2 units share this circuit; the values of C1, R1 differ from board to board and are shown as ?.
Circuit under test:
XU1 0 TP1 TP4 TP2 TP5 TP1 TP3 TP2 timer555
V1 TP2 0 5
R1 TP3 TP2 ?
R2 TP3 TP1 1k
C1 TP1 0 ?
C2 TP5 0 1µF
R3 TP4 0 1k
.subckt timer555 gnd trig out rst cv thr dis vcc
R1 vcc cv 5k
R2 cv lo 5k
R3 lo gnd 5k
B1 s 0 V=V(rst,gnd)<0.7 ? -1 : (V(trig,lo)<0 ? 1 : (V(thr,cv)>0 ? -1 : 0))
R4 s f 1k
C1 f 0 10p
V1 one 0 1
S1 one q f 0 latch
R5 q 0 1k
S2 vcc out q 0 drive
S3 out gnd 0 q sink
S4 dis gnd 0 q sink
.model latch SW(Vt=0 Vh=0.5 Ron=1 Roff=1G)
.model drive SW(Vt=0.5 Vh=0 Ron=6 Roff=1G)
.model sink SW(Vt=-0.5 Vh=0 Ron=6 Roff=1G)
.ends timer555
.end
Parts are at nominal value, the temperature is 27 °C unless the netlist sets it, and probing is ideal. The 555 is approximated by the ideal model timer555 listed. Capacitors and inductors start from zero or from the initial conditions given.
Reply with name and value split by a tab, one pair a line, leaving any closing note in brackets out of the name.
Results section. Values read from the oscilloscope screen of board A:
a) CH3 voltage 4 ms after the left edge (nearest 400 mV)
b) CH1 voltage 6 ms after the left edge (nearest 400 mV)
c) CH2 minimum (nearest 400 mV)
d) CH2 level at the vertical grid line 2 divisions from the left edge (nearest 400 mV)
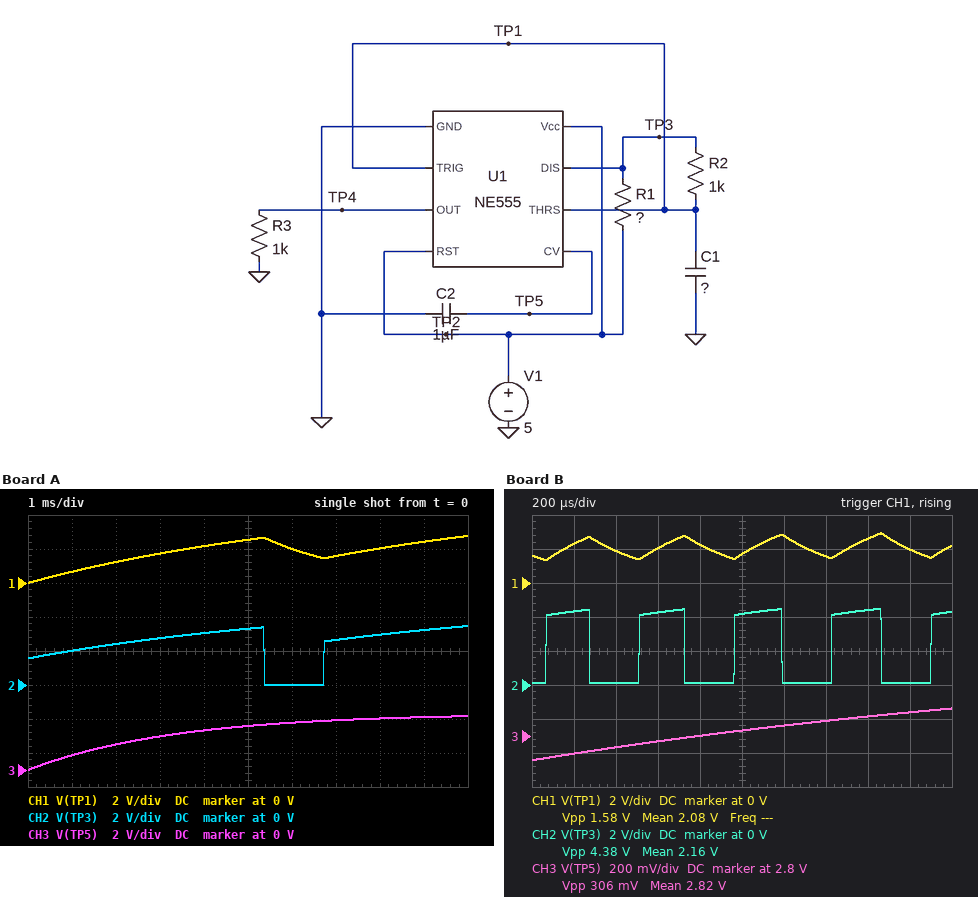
CH3 voltage 4 ms after the left edge	2.4 V
CH1 voltage 6 ms after the left edge	2.0 V
CH2 minimum	0 V
CH2 level at the vertical grid line 2 divisions from the left edge	2.4 V
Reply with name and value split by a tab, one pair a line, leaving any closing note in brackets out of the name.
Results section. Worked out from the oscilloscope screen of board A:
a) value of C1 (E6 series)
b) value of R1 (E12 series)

value of C1	2.2 µF
value of R1	2.2 kΩ
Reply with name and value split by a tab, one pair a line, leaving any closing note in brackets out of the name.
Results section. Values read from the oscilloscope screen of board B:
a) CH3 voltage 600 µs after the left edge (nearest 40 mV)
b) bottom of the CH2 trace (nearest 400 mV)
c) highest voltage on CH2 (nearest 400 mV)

CH3 voltage 600 µs after the left edge	2.76 V
bottom of the CH2 trace	0 V
highest voltage on CH2	4.4 V
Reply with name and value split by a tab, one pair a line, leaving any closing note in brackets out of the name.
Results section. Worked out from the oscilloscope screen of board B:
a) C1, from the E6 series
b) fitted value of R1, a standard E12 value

C1, from the E6 series	330 nF
fitted value of R1, a standard E12 value	330 Ω
